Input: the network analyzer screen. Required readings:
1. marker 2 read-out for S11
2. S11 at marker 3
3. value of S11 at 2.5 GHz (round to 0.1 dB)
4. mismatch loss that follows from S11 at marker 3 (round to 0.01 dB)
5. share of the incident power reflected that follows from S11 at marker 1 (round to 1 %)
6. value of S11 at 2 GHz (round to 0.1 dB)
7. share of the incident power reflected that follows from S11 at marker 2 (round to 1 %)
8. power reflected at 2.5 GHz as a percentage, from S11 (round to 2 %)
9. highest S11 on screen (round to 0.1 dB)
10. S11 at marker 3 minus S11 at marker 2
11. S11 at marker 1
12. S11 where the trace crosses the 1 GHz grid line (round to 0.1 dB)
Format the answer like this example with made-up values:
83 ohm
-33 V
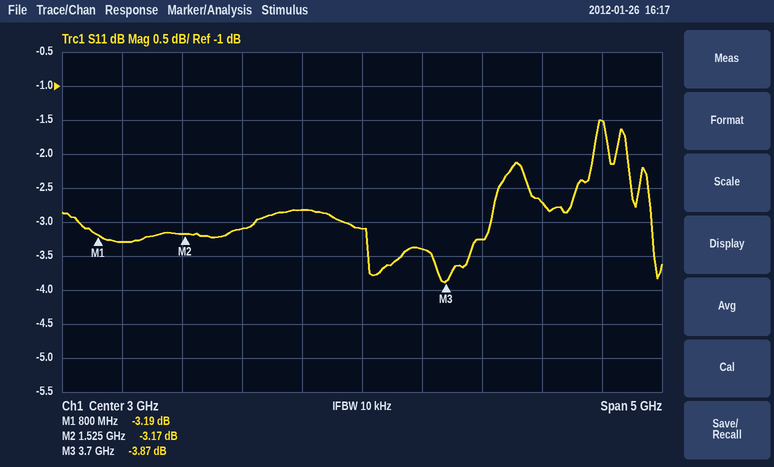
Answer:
-3.17 dB
-3.87 dB
-2.8 dB
2.29 dB
48 %
-3.1 dB
48 %
52 %
-1.5 dB
-0.70 dB
-3.19 dB
-3.3 dB
